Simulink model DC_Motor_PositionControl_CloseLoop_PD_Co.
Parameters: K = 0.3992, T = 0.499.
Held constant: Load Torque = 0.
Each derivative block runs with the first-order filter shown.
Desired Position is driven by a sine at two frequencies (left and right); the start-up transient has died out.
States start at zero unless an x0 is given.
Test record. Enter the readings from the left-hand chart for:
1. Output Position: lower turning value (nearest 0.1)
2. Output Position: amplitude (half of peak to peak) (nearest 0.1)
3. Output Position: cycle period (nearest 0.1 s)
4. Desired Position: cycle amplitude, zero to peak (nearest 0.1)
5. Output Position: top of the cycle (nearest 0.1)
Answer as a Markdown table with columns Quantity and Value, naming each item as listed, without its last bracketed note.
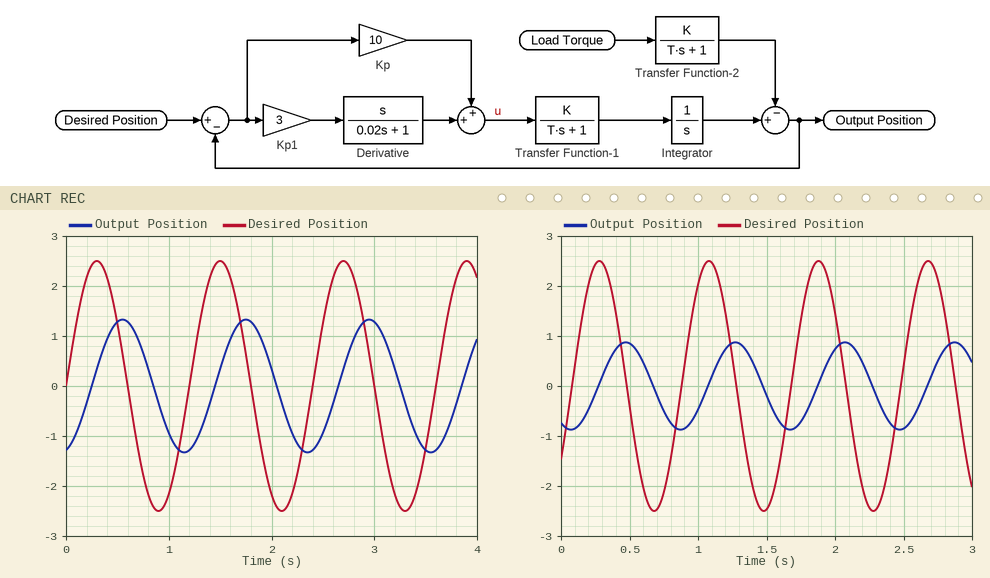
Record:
| Quantity | Value |
|---|---|
| Output Position: lower turning value | -1.3 |
| Output Position: amplitude (half of peak to peak) | 1.3 |
| Output Position: cycle period | 1.2 s |
| Desired Position: cycle amplitude, zero to peak | 2.5 |
| Output Position: top of the cycle | 1.3 |
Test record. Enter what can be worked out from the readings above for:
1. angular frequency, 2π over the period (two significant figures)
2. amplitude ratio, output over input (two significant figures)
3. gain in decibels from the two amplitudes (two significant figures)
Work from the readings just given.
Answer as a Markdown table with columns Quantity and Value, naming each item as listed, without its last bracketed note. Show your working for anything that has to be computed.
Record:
| Quantity | Value |
|---|---|
| angular frequency, 2π over the period | 2π / 1.2 = 5.2 rad/s |
| amplitude ratio, output over input | 1.3 / 2.5 = 0.52 |
| gain in decibels from the two amplitudes | 20 log10(1.3 / 2.5) = -5.7 dB |
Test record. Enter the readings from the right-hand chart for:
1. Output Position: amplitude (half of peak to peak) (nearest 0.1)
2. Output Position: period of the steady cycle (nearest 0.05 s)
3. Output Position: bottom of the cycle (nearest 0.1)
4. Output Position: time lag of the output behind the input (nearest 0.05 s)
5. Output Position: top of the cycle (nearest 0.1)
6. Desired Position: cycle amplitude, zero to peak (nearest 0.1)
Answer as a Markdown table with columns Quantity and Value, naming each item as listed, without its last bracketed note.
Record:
| Quantity | Value |
|---|---|
| Output Position: amplitude (half of peak to peak) | 0.9 |
| Output Position: period of the steady cycle | 0.80 s |
| Output Position: bottom of the cycle | -0.9 |
| Output Position: time lag of the output behind the input | 0.20 s |
| Output Position: top of the cycle | 0.9 |
| Desired Position: cycle amplitude, zero to peak | 2.5 |
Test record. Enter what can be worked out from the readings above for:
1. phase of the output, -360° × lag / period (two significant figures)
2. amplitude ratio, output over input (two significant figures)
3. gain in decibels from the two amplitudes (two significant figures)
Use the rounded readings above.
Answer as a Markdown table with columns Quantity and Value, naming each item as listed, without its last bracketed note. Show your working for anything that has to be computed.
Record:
| Quantity | Value |
|---|---|
| phase of the output, -360° × lag / period | -360 × 0.2 / 0.8 = -90° |
| amplitude ratio, output over input | 0.9 / 2.5 = 0.36 |
| gain in decibels from the two amplitudes | 20 log10(0.9 / 2.5) = -8.9 dB |
